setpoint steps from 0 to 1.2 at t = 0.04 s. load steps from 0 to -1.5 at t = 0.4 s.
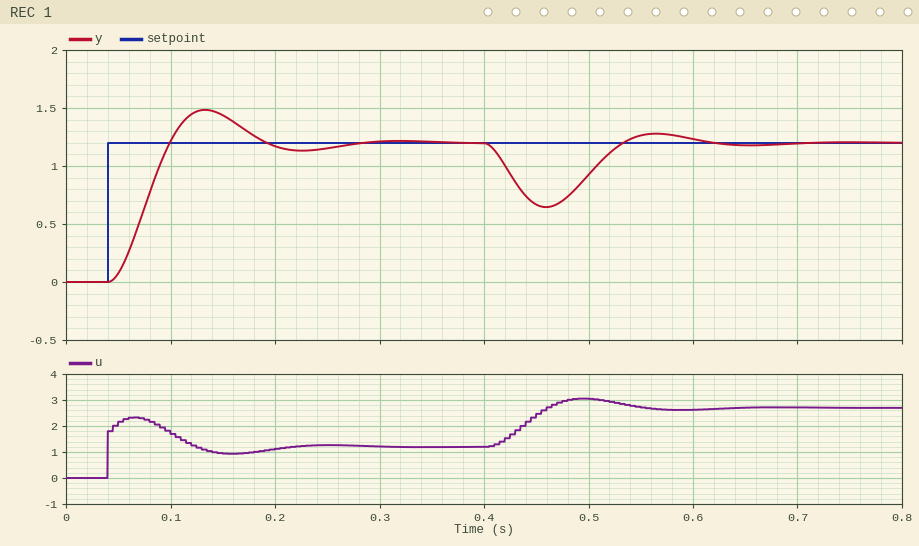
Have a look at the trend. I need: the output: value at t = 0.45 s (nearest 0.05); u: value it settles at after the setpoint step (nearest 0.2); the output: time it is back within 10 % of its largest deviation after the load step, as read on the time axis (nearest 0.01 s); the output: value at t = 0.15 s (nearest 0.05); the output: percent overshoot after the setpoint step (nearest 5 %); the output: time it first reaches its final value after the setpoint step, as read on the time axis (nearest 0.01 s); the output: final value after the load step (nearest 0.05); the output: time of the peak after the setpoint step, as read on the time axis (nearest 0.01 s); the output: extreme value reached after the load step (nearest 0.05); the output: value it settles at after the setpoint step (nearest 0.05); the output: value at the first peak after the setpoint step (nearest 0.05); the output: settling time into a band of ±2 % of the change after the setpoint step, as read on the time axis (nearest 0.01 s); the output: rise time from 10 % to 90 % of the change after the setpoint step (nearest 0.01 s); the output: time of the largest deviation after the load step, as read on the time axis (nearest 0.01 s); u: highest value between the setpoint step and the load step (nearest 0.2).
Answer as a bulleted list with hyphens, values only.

- 0.65
- 1.2
- 0.59 s
- 1.45
- 25 %
- 0.10 s
- 1.20
- 0.13 s
- 0.65
- 1.20
- 1.50
- 0.27 s
- 0.04 s
- 0.46 s
- 2.4
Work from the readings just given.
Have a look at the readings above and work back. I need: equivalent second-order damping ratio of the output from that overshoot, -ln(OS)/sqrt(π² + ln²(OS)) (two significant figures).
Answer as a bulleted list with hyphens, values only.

- 0.40
